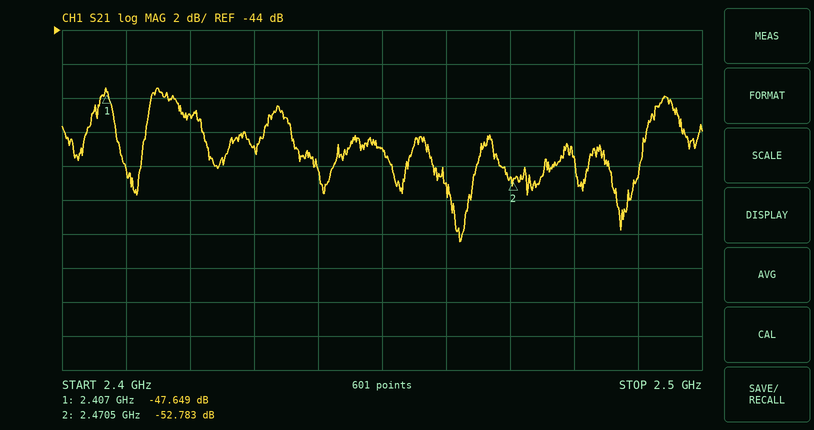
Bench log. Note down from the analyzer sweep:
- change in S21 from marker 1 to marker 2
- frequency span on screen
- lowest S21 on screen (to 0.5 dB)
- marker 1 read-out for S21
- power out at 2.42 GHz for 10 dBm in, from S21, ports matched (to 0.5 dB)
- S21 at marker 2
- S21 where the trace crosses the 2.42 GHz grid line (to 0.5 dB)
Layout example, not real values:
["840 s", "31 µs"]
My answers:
["-5.134 dB", "100 MHz", "-56.5 dB", "-47.649 dB", "-39.0 dBm", "-52.783 dB", "-49.0 dB"]
